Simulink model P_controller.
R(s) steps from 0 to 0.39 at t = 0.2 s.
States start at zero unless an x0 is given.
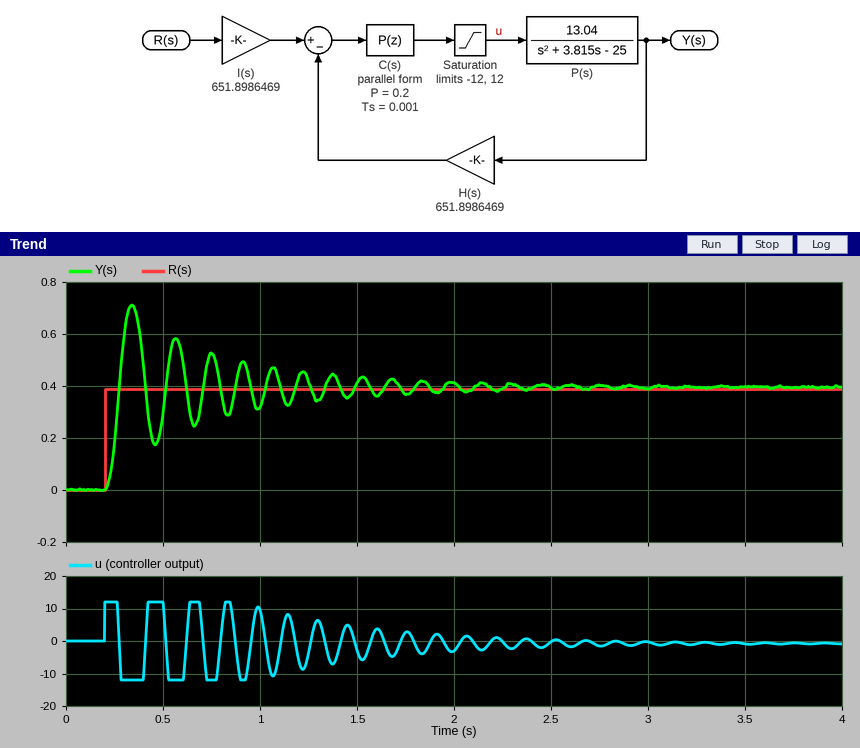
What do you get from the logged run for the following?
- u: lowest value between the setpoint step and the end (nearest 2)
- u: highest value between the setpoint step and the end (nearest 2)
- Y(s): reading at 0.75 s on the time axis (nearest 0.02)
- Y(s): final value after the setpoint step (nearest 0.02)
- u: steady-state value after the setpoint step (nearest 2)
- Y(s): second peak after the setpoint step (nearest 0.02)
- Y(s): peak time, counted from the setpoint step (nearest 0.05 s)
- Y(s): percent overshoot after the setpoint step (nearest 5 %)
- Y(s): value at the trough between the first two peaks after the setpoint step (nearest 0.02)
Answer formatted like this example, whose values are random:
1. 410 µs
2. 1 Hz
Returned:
1. -12
2. 12
3. 0.52
4. 0.40
5. 0
6. 0.58
7. 0.15 s
8. 80 %
9. 0.18
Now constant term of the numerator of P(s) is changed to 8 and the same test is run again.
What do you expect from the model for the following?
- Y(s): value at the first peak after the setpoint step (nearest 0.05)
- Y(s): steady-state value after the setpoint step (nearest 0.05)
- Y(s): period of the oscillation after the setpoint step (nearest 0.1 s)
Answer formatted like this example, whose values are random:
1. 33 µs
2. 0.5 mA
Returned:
1. 0.70
2. 0.40
3. 0.3 s
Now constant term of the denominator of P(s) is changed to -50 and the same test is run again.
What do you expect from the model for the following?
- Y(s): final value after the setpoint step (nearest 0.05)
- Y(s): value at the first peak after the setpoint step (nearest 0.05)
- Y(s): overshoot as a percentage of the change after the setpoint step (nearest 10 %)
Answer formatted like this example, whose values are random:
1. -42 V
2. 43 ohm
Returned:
1. 0.40
2. 0.75
3. 90 %
